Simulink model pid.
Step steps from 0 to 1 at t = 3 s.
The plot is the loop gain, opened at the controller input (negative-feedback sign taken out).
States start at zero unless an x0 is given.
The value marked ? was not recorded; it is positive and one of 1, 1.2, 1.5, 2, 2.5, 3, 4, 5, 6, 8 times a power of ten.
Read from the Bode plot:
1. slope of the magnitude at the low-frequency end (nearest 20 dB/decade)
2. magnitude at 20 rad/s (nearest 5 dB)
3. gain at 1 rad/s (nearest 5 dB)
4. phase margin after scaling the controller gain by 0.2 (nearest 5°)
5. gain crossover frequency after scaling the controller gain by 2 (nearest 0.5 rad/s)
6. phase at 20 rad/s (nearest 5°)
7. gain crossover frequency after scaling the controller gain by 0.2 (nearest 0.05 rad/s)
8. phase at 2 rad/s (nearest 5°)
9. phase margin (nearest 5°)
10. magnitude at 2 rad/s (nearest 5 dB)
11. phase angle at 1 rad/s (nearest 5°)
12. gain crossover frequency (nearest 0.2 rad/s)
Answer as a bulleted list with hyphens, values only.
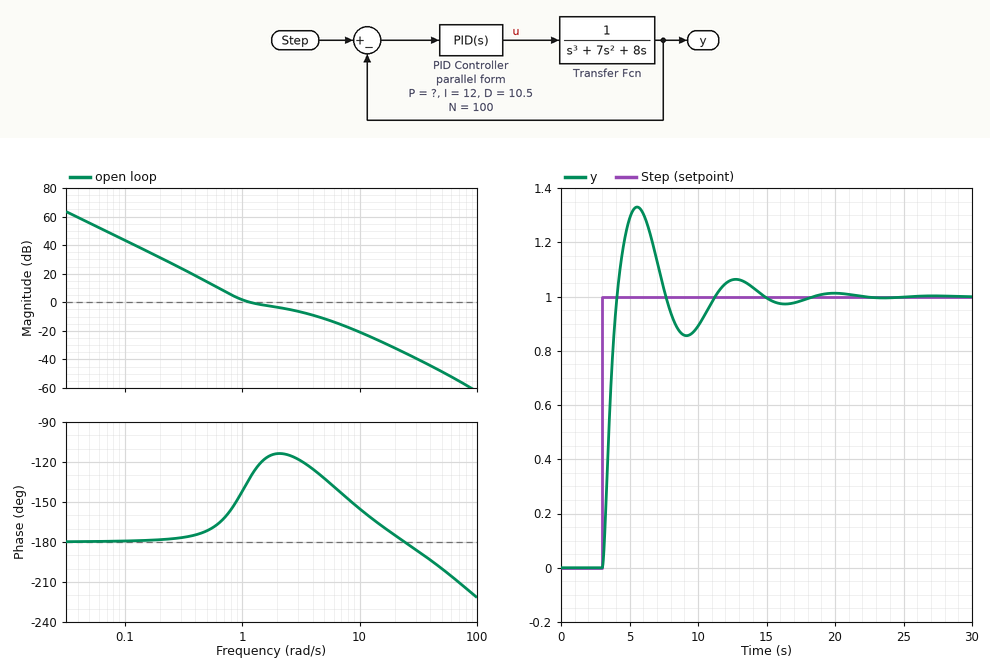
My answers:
- -40 dB/decade
- -30 dB
- 0 dB
- 10°
- 3.0 rad/s
- -175°
- 0.50 rad/s
- -115°
- 50°
- -5 dB
- -140°
- 1.2 rad/s
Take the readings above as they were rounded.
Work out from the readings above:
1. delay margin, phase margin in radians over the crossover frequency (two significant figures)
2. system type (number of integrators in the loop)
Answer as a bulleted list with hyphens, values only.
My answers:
- 0.73 s
- 2
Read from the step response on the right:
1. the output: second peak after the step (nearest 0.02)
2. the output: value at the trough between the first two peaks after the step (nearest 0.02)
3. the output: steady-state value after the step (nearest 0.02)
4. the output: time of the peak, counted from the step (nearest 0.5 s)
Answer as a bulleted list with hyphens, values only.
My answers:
- 1.06
- 0.86
- 1.00
- 2.5 s
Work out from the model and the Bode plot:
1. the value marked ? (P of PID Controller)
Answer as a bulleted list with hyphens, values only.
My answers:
- 12
